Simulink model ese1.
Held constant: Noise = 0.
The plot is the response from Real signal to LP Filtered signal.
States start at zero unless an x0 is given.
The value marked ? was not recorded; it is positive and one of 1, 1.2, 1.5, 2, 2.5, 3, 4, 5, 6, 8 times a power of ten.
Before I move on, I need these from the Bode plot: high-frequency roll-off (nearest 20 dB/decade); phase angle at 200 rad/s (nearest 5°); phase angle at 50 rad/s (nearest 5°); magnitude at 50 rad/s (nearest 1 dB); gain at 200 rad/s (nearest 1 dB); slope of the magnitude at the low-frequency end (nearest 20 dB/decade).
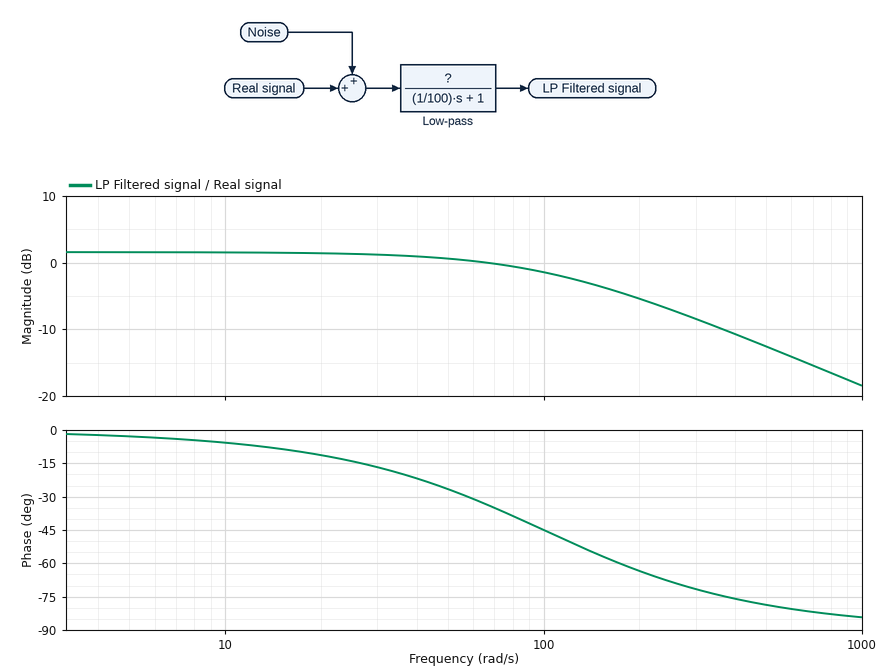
-20 dB/decade
-65°
-25°
1 dB
-5 dB
0 dB/decade
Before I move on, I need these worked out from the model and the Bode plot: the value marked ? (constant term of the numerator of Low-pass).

1.2
